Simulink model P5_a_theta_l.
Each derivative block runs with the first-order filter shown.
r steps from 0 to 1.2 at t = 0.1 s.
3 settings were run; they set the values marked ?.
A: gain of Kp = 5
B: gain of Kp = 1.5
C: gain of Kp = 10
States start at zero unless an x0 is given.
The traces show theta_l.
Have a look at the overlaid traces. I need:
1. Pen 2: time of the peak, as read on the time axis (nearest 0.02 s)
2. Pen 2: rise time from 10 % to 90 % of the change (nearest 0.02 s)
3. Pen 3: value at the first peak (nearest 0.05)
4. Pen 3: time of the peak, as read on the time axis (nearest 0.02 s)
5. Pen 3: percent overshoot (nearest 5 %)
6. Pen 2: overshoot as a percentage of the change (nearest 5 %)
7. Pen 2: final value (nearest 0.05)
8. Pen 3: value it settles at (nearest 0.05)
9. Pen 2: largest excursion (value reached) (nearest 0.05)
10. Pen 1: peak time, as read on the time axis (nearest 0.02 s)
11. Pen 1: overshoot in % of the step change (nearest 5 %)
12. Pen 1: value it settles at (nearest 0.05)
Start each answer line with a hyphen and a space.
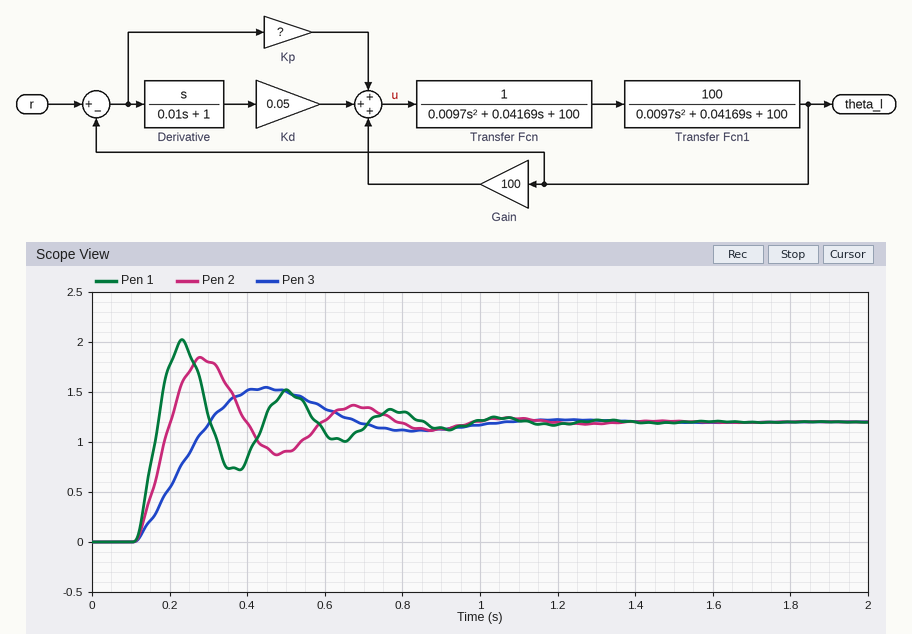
- 0.28 s
- 0.06 s
- 1.55
- 0.44 s
- 30 %
- 55 %
- 1.20
- 1.20
- 1.85
- 0.24 s
- 70 %
- 1.20
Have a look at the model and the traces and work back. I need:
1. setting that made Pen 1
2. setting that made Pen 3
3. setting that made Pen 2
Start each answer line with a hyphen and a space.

- C
- B
- A
